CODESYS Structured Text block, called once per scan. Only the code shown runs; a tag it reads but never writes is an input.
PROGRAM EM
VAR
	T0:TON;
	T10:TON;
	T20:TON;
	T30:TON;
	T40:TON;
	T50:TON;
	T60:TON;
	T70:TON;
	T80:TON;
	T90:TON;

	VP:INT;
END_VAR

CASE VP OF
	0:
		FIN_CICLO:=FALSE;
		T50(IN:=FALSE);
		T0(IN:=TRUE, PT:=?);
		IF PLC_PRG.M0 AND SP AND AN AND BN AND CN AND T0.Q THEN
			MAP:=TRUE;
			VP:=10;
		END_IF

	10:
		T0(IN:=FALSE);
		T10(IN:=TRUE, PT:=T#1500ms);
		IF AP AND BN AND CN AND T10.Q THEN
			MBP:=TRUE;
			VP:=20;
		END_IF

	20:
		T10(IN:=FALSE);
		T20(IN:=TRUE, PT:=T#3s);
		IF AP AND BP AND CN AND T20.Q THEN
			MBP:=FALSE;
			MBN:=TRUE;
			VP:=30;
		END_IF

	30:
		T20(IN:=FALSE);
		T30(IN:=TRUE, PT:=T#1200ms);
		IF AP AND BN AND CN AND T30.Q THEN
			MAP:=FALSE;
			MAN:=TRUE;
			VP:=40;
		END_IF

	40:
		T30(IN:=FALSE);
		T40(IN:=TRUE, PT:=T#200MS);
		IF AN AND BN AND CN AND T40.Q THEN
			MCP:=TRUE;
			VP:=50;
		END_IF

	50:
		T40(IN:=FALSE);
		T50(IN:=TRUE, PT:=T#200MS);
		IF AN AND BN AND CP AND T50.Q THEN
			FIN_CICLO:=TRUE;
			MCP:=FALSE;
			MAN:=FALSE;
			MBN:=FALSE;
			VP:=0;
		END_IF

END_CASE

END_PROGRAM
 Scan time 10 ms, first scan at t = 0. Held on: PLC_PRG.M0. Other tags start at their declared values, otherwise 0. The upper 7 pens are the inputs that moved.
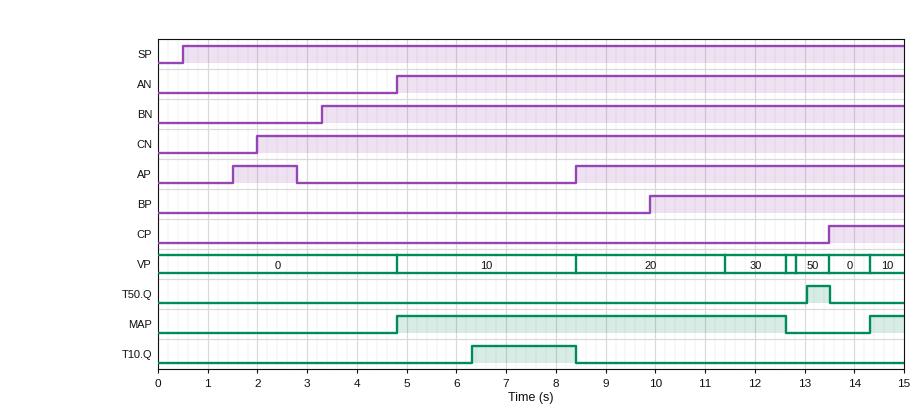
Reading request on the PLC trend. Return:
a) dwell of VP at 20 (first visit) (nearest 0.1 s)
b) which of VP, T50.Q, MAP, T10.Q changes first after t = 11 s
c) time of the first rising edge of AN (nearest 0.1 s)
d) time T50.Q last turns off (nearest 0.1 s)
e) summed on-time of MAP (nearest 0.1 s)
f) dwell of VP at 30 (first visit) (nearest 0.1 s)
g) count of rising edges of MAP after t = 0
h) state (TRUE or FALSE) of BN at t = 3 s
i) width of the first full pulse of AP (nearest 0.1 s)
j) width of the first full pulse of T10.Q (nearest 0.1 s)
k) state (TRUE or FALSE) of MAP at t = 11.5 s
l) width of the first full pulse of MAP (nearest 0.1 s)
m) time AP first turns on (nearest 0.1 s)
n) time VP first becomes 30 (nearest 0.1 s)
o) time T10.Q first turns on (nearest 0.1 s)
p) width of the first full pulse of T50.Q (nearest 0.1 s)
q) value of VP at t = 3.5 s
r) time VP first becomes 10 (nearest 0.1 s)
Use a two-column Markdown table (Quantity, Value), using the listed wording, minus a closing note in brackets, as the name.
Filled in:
| Quantity | Value |
|---|---|
| dwell of VP at 20 (first visit) | 3.0 s |
| which of VP, T50.Q, MAP, T10.Q changes first after t = 11 s | VP |
| time of the first rising edge of AN | 4.8 s |
| time T50.Q last turns off | 13.5 s |
| summed on-time of MAP | 8.5 s |
| dwell of VP at 30 (first visit) | 1.2 s |
| count of rising edges of MAP after t = 0 | 2 |
| state (TRUE or FALSE) of BN at t = 3 s | FALSE |
| width of the first full pulse of AP | 1.3 s |
| width of the first full pulse of T10.Q | 2.1 s |
| state (TRUE or FALSE) of MAP at t = 11.5 s | TRUE |
| width of the first full pulse of MAP | 7.8 s |
| time AP first turns on | 1.5 s |
| time VP first becomes 30 | 11.4 s |
| time T10.Q first turns on | 6.3 s |
| width of the first full pulse of T50.Q | 0.5 s |
| value of VP at t = 3.5 s | 0 |
| time VP first becomes 10 | 4.8 s |
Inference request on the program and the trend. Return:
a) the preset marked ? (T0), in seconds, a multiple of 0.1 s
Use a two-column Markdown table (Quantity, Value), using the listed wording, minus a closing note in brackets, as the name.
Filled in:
| Quantity | Value |
|---|---|
| the preset marked ? (T0), in seconds, a multiple of 0.1 s | 0.8 s |
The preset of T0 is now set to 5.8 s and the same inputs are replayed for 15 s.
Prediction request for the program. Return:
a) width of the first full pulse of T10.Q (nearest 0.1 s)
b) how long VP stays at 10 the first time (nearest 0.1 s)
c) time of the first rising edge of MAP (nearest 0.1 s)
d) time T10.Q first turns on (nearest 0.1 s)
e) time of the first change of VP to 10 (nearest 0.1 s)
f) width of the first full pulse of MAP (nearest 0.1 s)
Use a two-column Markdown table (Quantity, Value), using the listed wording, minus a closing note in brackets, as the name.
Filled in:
| Quantity | Value |
|---|---|
| width of the first full pulse of T10.Q | 1.1 s |
| how long VP stays at 10 the first time | 2.6 s |
| time of the first rising edge of MAP | 5.8 s |
| time T10.Q first turns on | 7.3 s |
| time of the first change of VP to 10 | 5.8 s |
| width of the first full pulse of MAP | 6.8 s |
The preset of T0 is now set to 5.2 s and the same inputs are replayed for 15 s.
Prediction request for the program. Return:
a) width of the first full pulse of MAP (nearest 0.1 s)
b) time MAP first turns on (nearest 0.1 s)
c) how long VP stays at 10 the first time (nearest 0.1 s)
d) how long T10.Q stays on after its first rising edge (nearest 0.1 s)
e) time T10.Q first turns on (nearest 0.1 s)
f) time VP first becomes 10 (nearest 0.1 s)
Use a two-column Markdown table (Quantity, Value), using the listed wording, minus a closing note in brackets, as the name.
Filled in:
| Quantity | Value |
|---|---|
| width of the first full pulse of MAP | 7.4 s |
| time MAP first turns on | 5.2 s |
| how long VP stays at 10 the first time | 3.2 s |
| how long T10.Q stays on after its first rising edge | 1.7 s |
| time T10.Q first turns on | 6.7 s |
| time VP first becomes 10 | 5.2 s |
